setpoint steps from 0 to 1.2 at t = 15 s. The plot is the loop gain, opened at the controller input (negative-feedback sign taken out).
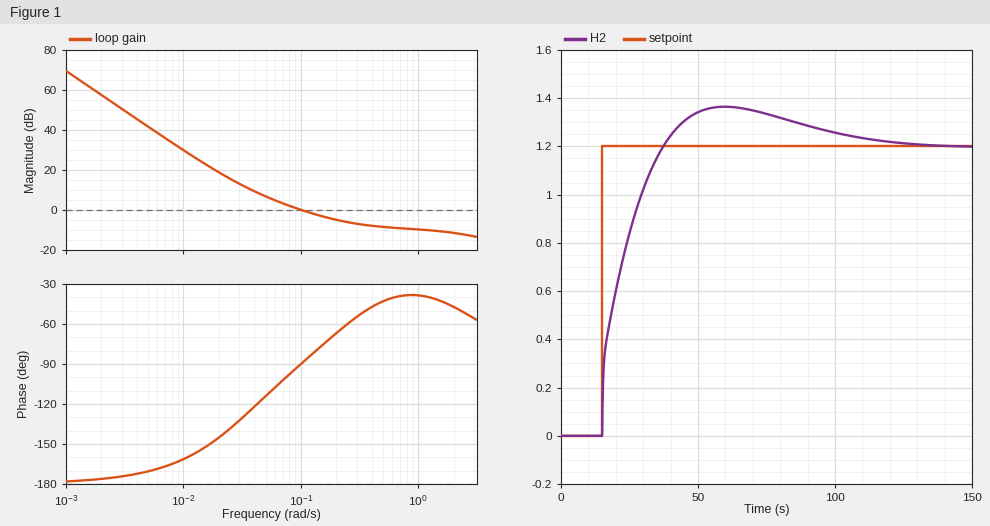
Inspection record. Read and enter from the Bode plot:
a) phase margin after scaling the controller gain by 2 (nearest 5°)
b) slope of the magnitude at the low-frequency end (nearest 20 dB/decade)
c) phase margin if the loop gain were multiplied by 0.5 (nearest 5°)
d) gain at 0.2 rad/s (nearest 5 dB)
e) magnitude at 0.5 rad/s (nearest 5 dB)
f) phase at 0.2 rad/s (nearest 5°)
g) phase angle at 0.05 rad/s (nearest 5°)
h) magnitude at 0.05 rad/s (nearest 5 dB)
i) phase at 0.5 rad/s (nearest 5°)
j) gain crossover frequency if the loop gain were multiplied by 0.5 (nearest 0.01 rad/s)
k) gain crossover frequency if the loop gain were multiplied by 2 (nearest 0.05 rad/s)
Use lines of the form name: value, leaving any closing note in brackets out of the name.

phase margin after scaling the controller gain by 2: 120°
slope of the magnitude at the low-frequency end: -40 dB/decade
phase margin if the loop gain were multiplied by 0.5: 70°
gain at 0.2 rad/s: -5 dB
magnitude at 0.5 rad/s: -10 dB
phase at 0.2 rad/s: -65°
phase angle at 0.05 rad/s: -115°
magnitude at 0.05 rad/s: 5 dB
phase at 0.5 rad/s: -45°
gain crossover frequency if the loop gain were multiplied by 0.5: 0.05 rad/s
gain crossover frequency if the loop gain were multiplied by 2: 0.25 rad/s
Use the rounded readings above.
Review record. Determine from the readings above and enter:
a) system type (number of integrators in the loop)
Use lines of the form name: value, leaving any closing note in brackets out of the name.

system type: 2
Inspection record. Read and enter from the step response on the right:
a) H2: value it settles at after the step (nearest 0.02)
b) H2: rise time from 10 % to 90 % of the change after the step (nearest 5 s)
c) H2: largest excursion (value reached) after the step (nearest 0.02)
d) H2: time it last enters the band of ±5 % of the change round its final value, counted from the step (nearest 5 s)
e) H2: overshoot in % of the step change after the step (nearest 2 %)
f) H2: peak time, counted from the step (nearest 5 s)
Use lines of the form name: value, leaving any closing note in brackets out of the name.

H2: value it settles at after the step: 1.20
H2: rise time from 10 % to 90 % of the change after the step: 15 s
H2: largest excursion (value reached) after the step: 1.36
H2: time it last enters the band of ±5 % of the change round its final value, counted from the step: 85 s
H2: overshoot in % of the step change after the step: 14 %
H2: peak time, counted from the step: 45 s
